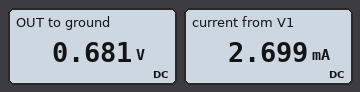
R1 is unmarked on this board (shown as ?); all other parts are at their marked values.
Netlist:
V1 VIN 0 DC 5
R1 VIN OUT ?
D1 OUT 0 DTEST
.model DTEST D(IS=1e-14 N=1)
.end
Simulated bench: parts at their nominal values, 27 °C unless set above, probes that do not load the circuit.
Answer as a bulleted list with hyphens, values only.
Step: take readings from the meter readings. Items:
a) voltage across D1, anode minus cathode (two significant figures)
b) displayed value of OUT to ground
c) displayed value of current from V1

- 680 mV
- 0.681 V
- 2.699 mA
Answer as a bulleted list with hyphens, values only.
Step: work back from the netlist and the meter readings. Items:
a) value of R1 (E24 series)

- 1.6 kΩ
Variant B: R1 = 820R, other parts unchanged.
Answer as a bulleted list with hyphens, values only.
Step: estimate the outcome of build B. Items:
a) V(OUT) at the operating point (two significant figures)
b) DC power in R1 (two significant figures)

- 700 mV
- 23 mW
